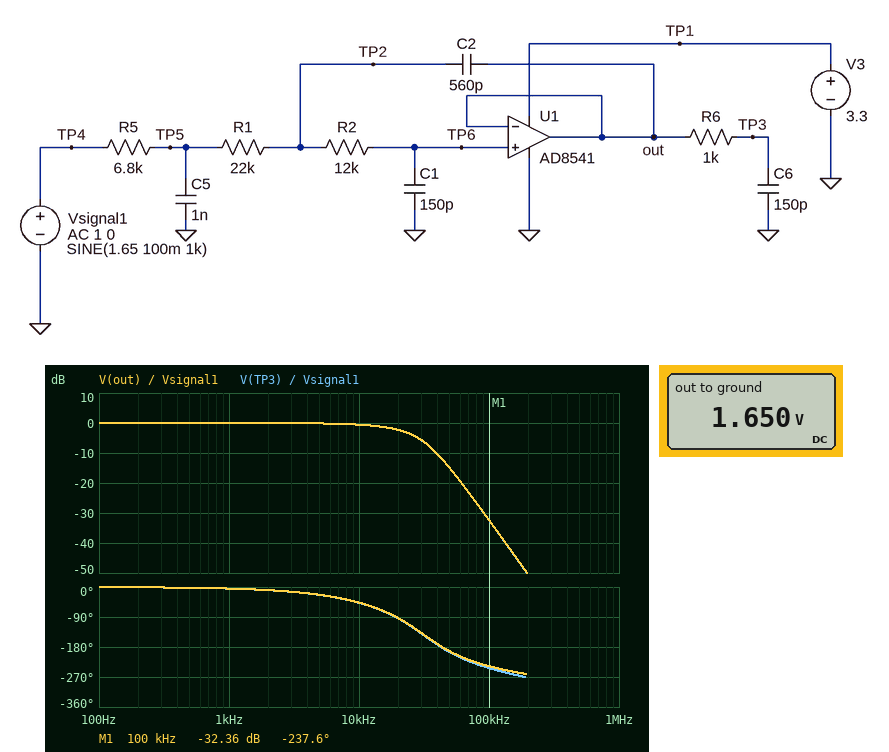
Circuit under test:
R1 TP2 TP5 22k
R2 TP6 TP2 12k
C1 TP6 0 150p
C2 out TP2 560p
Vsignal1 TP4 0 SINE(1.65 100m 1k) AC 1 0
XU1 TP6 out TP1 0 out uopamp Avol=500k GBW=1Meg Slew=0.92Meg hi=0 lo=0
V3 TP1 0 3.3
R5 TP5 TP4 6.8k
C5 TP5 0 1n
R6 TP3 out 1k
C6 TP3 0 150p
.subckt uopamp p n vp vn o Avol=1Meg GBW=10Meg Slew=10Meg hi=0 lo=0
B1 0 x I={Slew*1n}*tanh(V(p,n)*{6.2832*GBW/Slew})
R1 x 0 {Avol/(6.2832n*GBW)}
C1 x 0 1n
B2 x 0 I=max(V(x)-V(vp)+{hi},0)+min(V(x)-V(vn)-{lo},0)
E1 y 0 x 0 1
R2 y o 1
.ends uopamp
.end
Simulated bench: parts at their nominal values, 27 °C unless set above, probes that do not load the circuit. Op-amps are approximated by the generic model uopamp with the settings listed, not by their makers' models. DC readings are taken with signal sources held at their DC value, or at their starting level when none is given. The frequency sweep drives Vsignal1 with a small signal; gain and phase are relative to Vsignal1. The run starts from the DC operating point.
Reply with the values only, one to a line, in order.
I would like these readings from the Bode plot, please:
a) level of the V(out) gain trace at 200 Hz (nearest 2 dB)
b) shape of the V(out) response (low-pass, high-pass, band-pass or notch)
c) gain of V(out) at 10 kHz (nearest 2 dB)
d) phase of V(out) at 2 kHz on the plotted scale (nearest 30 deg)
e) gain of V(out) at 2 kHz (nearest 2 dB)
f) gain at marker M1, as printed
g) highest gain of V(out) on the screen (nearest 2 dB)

0 dB
low-pass
0 dB
0 deg
0 dB
-32.36 dB
0 dB
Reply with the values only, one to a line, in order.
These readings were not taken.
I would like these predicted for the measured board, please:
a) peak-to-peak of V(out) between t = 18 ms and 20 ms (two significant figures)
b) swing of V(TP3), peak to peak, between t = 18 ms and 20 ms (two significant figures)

200 mV
200 mV
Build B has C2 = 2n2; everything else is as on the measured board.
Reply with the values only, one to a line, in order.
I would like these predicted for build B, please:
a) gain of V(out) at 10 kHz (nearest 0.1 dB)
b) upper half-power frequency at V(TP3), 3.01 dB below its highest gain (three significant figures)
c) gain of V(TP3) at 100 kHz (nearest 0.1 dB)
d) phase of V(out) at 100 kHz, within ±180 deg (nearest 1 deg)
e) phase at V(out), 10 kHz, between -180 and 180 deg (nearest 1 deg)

2.5 dB
16.9 kHz
-44.4 dB
107 deg
-61 deg
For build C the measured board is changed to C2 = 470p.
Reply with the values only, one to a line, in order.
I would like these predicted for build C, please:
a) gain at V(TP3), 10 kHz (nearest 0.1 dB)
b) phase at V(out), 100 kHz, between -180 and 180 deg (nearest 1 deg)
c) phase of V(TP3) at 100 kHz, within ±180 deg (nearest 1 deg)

-0.7 dB
126 deg
121 deg
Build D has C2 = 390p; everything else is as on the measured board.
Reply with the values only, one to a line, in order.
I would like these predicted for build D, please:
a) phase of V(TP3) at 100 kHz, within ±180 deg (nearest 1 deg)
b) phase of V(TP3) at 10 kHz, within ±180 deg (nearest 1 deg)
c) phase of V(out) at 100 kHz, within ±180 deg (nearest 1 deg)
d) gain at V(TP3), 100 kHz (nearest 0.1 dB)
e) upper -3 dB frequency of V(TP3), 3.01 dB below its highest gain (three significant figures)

126 deg
-46 deg
131 deg
-29.5 dB
20.3 kHz
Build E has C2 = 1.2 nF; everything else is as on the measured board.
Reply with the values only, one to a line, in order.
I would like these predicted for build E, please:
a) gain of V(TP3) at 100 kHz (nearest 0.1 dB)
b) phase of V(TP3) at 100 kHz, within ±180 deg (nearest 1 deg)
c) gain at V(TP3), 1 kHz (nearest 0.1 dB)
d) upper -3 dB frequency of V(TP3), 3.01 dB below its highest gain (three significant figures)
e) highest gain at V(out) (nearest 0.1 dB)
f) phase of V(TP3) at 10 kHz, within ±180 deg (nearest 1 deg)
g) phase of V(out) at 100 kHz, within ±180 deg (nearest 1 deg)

-39.0 dB
106 deg
0 dB
22.1 kHz
0.7 dB
-52 deg
111 deg
